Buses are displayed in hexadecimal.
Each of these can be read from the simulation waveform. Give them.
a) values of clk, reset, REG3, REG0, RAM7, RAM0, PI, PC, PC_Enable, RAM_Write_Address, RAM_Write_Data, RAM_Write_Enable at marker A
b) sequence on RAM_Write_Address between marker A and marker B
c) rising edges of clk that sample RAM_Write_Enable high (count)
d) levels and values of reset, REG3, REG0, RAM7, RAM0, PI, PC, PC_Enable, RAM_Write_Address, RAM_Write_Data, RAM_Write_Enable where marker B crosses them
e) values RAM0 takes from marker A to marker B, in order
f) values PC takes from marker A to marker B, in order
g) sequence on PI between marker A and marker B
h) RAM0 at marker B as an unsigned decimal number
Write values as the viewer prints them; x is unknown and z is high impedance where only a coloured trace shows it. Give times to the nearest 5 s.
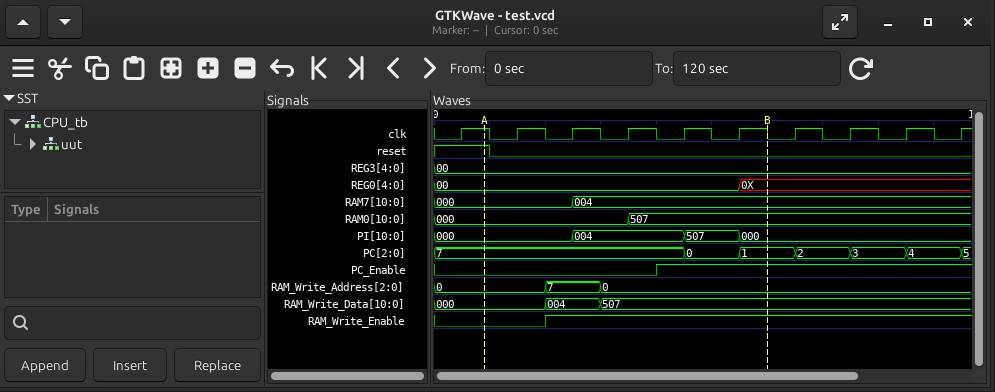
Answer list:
clk=1, reset=1, REG3=00, REG0=00, RAM7=000, RAM0=000, PI=000, PC=7, PC_Enable=0, RAM_Write_Address=0, RAM_Write_Data=000, RAM_Write_Enable=0
0, 7, 0
8
reset=0, REG3=00, REG0=0X, RAM7=004, RAM0=507, PI=000, PC=1, PC_Enable=1, RAM_Write_Address=0, RAM_Write_Data=507, RAM_Write_Enable=1
000, 507
7, 0, 1
000, 004, 507, 000
1287
